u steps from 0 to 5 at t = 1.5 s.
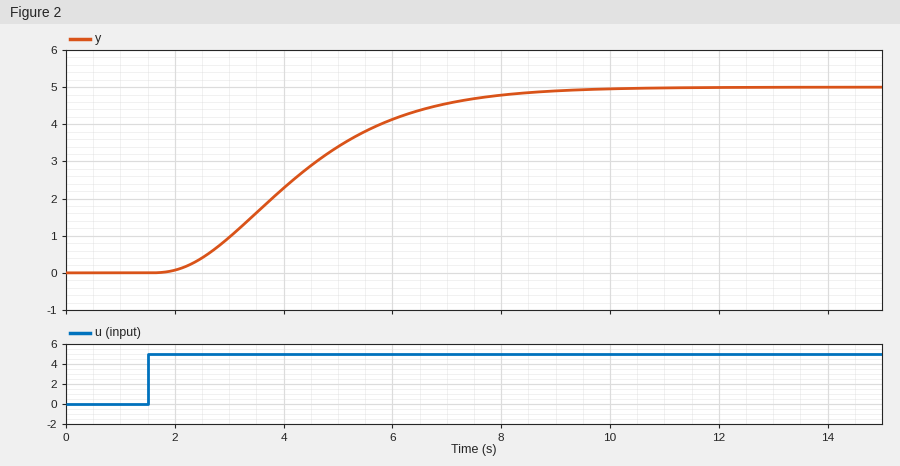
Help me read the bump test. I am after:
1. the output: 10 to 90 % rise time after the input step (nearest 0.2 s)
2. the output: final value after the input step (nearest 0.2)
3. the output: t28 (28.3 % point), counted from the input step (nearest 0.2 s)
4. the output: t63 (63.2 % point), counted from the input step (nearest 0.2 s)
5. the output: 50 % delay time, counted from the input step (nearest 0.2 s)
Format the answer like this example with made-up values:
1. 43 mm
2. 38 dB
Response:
1. 4.2 s
2. 5.0
3. 1.8 s
4. 3.2 s
5. 2.6 s
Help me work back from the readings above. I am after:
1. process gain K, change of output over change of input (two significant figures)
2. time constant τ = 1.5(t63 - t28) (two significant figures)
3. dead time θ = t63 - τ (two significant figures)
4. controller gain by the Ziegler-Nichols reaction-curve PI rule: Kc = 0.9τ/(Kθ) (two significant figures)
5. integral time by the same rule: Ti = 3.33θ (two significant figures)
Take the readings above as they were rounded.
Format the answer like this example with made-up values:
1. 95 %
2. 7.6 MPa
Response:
1. 1.0
2. 2.1 s
3. 1.1 s
4. 1.7
5. 3.7 s
